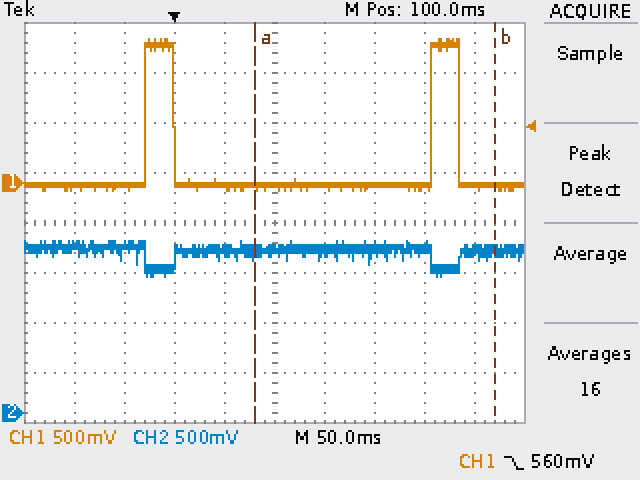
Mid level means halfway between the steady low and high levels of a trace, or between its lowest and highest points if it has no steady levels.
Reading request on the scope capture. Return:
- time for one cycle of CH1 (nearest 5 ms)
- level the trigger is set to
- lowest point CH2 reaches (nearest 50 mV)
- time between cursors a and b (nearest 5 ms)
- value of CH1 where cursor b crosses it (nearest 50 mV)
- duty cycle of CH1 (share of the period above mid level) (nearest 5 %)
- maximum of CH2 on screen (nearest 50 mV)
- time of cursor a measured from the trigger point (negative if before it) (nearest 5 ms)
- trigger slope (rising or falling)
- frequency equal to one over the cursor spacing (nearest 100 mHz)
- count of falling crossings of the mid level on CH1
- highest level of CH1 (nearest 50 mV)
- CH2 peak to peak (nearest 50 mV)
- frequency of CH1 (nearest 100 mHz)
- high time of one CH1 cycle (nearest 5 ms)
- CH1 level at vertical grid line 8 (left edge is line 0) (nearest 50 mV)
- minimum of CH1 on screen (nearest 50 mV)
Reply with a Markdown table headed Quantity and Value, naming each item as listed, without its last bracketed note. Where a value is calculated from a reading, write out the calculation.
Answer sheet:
| Quantity | Value |
|---|---|
| time for one cycle of CH1 | 285 ms |
| level the trigger is set to | 560 mV |
| lowest point CH2 reaches | 1.35 V |
| time between cursors a and b | 240 ms |
| value of CH1 where cursor b crosses it | -50 mV |
| duty cycle of CH1 (share of the period above mid level) | 30 ms / 285 ms ≈ 10 % |
| maximum of CH2 on screen | 1.70 V |
| time of cursor a measured from the trigger point (negative if before it) | +80 ms |
| trigger slope | falling |
| frequency equal to one over the cursor spacing | 1 / 240 ms ≈ 4.2 Hz |
| count of falling crossings of the mid level on CH1 | 2 |
| highest level of CH1 | 1.45 V |
| CH2 peak to peak | 1.70 V − (1.35 V) = 350 mV |
| frequency of CH1 | 1 / 285 ms ≈ 3.5 Hz |
| high time of one CH1 cycle | 30 ms |
| CH1 level at vertical grid line 8 (left edge is line 0) | -50 mV |
| minimum of CH1 on screen | -100 mV |
